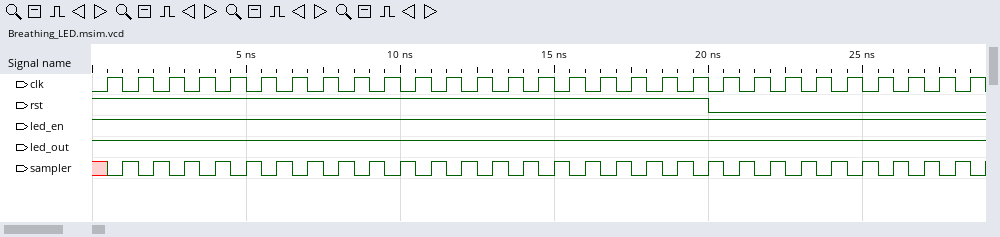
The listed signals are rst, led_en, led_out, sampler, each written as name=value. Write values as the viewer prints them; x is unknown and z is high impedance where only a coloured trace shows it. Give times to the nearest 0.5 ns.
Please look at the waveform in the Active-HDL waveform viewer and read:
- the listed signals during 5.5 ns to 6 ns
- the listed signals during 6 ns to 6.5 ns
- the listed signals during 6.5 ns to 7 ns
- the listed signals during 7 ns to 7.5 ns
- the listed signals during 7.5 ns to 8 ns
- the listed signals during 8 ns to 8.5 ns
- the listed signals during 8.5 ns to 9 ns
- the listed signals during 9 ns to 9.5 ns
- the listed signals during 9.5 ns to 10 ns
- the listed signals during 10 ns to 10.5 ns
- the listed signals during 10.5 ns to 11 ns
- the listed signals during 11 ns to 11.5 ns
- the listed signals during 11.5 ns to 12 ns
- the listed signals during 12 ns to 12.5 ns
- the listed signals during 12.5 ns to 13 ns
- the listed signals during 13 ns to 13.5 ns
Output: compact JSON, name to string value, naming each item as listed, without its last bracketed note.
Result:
{"the listed signals during 5.5 ns to 6 ns": "rst=1, led_en=1, led_out=1, sampler=0", "the listed signals during 6 ns to 6.5 ns": "rst=1, led_en=1, led_out=1, sampler=1", "the listed signals during 6.5 ns to 7 ns": "rst=1, led_en=1, led_out=1, sampler=0", "the listed signals during 7 ns to 7.5 ns": "rst=1, led_en=1, led_out=1, sampler=1", "the listed signals during 7.5 ns to 8 ns": "rst=1, led_en=1, led_out=1, sampler=0", "the listed signals during 8 ns to 8.5 ns": "rst=1, led_en=1, led_out=1, sampler=1", "the listed signals during 8.5 ns to 9 ns": "rst=1, led_en=1, led_out=1, sampler=0", "the listed signals during 9 ns to 9.5 ns": "rst=1, led_en=1, led_out=1, sampler=1", "the listed signals during 9.5 ns to 10 ns": "rst=1, led_en=1, led_out=1, sampler=0", "the listed signals during 10 ns to 10.5 ns": "rst=1, led_en=1, led_out=1, sampler=1", "the listed signals during 10.5 ns to 11 ns": "rst=1, led_en=1, led_out=1, sampler=0", "the listed signals during 11 ns to 11.5 ns": "rst=1, led_en=1, led_out=1, sampler=1", "the listed signals during 11.5 ns to 12 ns": "rst=1, led_en=1, led_out=1, sampler=0", "the listed signals during 12 ns to 12.5 ns": "rst=1, led_en=1, led_out=1, sampler=1", "the listed signals during 12.5 ns to 13 ns": "rst=1, led_en=1, led_out=1, sampler=0", "the listed signals during 13 ns to 13.5 ns": "rst=1, led_en=1, led_out=1, sampler=1"}
